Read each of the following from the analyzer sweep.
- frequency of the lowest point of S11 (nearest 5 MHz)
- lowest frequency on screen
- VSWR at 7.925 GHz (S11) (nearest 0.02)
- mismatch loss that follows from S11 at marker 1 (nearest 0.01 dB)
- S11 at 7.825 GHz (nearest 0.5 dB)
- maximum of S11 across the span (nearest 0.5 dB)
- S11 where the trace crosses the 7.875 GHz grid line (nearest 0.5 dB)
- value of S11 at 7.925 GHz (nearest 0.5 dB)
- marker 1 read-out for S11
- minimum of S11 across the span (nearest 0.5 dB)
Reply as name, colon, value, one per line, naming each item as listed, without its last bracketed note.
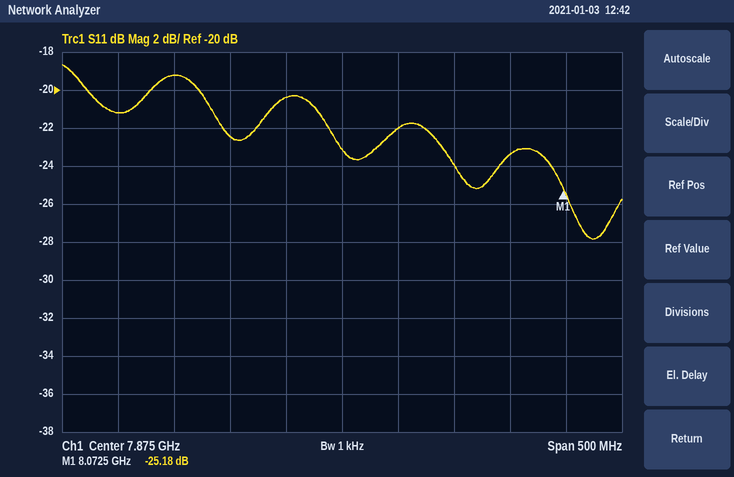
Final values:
frequency of the lowest point of S11: 8.100 GHz
lowest frequency on screen: 7.625 GHz
VSWR at 7.925 GHz (S11): 1.18
mismatch loss that follows from S11 at marker 1: 0.01 dB
S11 at 7.825 GHz: -20.5 dB
maximum of S11 across the span: -18.5 dB
S11 where the trace crosses the 7.875 GHz grid line: -23.0 dB
value of S11 at 7.925 GHz: -22.0 dB
marker 1 read-out for S11: -25.18 dB
minimum of S11 across the span: -28.0 dB
